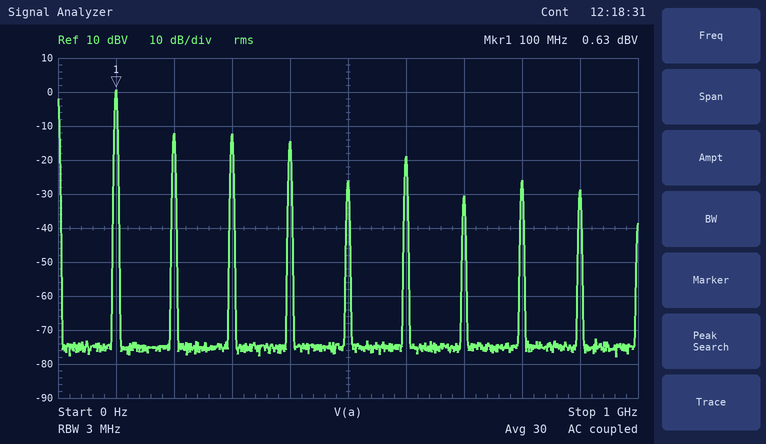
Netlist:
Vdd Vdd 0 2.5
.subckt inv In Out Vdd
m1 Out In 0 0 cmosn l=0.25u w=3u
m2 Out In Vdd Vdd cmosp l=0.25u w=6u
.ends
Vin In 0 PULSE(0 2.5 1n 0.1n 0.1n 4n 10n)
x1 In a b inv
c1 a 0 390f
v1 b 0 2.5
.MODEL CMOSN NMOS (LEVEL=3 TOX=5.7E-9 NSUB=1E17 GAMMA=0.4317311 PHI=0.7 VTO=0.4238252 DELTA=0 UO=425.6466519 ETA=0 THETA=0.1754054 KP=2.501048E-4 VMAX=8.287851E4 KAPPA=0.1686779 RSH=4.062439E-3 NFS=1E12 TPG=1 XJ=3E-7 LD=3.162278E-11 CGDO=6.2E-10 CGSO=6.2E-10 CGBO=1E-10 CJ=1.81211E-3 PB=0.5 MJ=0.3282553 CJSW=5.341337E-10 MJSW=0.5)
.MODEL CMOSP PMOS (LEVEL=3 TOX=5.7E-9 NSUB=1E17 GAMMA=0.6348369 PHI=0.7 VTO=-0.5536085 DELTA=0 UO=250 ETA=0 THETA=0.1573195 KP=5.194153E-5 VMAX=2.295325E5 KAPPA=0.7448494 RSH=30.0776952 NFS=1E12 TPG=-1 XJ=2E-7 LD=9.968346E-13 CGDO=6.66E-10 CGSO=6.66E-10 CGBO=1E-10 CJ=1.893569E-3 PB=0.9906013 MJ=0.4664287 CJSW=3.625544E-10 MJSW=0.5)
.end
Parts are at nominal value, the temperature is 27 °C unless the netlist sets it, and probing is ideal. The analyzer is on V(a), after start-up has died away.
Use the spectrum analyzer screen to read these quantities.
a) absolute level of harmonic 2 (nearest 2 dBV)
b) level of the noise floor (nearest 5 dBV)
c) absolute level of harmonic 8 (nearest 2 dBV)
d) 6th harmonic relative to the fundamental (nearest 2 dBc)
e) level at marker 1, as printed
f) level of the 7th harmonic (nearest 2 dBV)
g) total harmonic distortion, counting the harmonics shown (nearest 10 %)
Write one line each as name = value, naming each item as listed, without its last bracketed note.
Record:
absolute level of harmonic 2 = -12 dBV
level of the noise floor = -75 dBV
absolute level of harmonic 8 = -26 dBV
6th harmonic relative to the fundamental = -20 dBc
level at marker 1, as printed = 0.63 dBV
level of the 7th harmonic = -30 dBV
total harmonic distortion, counting the harmonics shown = 40 %
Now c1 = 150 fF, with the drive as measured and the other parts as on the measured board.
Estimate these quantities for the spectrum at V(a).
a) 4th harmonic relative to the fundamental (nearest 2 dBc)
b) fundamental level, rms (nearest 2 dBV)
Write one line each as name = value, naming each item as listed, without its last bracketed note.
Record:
4th harmonic relative to the fundamental = -14 dBc
fundamental level, rms = 0 dBV
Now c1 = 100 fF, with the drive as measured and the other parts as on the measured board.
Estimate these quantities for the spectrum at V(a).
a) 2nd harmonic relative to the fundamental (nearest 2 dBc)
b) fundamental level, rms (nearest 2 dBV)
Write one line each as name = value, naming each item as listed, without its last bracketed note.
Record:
2nd harmonic relative to the fundamental = -12 dBc
fundamental level, rms = 0 dBV
